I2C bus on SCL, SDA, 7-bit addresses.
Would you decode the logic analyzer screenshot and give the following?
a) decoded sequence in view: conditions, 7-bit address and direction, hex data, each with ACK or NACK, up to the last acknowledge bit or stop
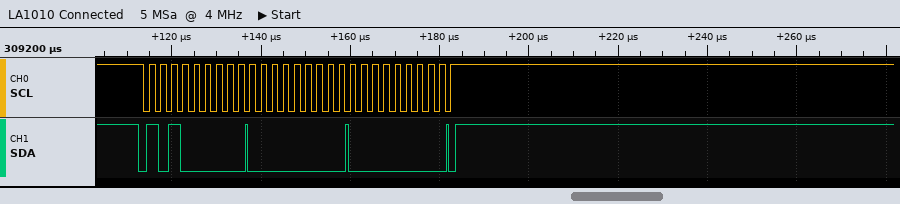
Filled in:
start, address 50 write ACK, 00 ACK, 00 ACK, stop
